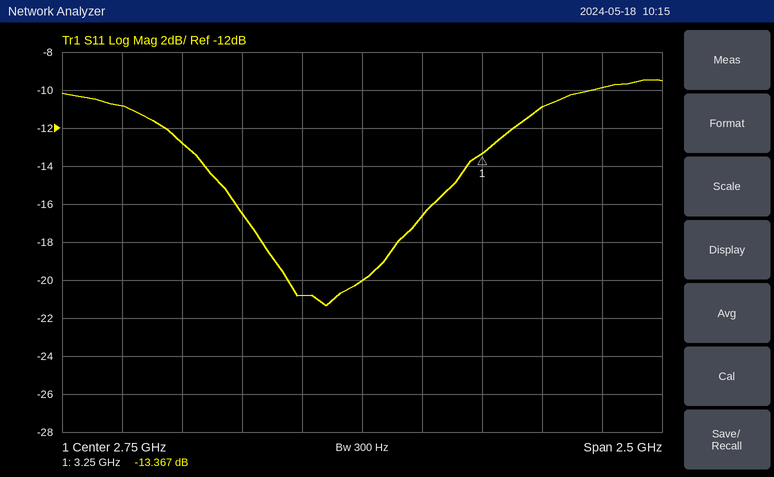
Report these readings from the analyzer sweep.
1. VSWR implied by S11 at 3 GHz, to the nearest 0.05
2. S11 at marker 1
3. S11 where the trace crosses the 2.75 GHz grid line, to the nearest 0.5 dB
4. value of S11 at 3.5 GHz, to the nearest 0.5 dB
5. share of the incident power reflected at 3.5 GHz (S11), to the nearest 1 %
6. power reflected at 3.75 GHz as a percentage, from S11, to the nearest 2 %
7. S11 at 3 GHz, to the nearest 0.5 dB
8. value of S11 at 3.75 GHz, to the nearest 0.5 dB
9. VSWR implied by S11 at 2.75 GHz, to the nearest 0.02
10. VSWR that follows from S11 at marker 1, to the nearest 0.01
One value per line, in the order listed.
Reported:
1.35
-13.367 dB
-20.0 dB
-11.0 dB
8 %
10 %
-16.5 dB
-10.0 dB
1.22
1.55
